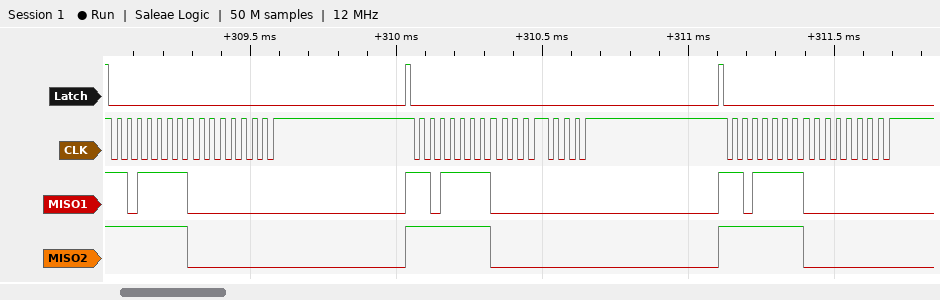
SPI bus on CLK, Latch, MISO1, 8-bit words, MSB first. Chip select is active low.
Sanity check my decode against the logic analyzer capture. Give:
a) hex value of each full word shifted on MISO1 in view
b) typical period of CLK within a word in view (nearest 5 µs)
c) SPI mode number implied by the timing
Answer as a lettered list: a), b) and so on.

a) DF, 00, DF, 00, DF, 00
b) 35 µs
c) 2
